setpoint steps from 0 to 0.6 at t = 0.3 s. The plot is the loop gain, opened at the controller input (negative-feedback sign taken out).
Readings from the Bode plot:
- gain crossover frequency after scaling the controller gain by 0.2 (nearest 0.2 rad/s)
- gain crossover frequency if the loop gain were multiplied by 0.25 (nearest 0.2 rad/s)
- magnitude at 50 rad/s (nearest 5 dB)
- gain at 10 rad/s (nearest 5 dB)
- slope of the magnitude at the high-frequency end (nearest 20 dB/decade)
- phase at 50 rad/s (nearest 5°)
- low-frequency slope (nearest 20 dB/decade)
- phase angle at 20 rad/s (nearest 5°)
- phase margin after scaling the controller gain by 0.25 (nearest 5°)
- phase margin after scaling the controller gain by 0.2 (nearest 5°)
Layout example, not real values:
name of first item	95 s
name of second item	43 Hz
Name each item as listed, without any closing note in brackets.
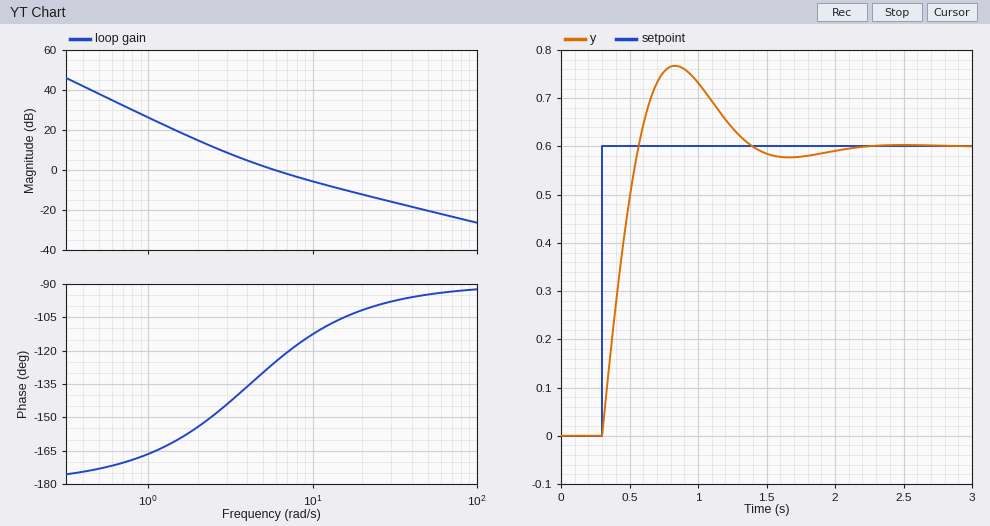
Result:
gain crossover frequency after scaling the controller gain by 0.2	2.2 rad/s
gain crossover frequency if the loop gain were multiplied by 0.25	2.4 rad/s
magnitude at 50 rad/s	-20 dB
gain at 10 rad/s	-5 dB
slope of the magnitude at the high-frequency end	-20 dB/decade
phase at 50 rad/s	-95°
low-frequency slope	-40 dB/decade
phase angle at 20 rad/s	-100°
phase margin after scaling the controller gain by 0.25	30°
phase margin after scaling the controller gain by 0.2	25°
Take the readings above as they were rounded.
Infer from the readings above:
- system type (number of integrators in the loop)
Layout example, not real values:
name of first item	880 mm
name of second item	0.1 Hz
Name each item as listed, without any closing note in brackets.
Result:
system type	2
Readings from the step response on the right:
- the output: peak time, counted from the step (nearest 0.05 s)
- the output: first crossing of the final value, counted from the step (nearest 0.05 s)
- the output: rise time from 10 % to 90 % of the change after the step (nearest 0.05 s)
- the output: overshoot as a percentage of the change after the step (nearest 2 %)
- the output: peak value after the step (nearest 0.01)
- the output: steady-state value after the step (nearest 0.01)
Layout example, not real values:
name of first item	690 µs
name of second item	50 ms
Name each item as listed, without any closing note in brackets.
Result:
the output: peak time, counted from the step	0.55 s
the output: first crossing of the final value, counted from the step	0.25 s
the output: rise time from 10 % to 90 % of the change after the step	0.20 s
the output: overshoot as a percentage of the change after the step	28 %
the output: peak value after the step	0.77
the output: steady-state value after the step	0.60
